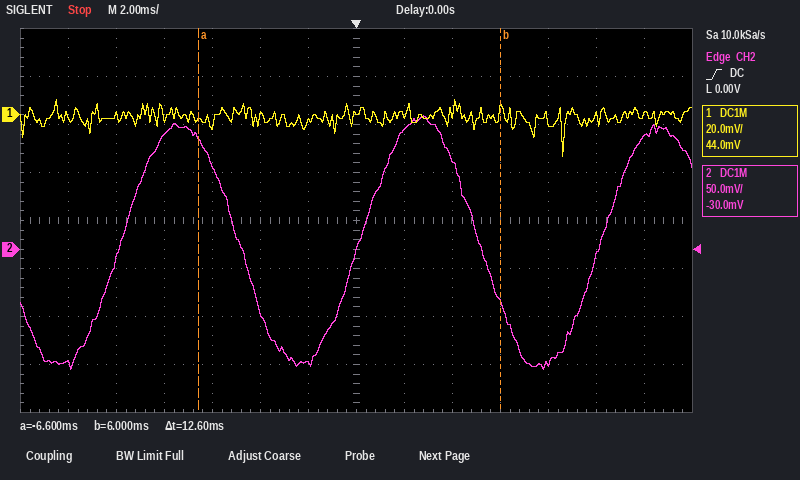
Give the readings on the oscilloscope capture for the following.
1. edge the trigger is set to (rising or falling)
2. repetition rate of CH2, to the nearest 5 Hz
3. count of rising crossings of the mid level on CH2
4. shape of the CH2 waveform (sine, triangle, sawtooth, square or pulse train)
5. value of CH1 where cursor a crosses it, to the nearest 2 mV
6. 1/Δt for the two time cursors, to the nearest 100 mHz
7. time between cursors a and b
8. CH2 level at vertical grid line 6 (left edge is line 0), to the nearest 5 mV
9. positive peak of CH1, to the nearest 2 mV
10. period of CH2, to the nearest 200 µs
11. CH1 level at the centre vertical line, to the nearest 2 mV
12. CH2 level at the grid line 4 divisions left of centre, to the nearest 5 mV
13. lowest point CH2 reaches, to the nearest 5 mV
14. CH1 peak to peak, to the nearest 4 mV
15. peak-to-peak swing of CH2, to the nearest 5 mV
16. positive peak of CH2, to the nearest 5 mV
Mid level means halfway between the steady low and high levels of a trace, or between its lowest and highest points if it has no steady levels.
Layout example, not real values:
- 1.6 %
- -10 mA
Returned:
- rising
- 100 Hz
- 3
- sine
- -2 mV
- 79.4 Hz
- 12.6 ms
- -120 mV
- 6 mV
- 10.0 ms
- 0 mV
- 120 mV
- -125 mV
- 24 mV
- 265 mV
- 140 mV
